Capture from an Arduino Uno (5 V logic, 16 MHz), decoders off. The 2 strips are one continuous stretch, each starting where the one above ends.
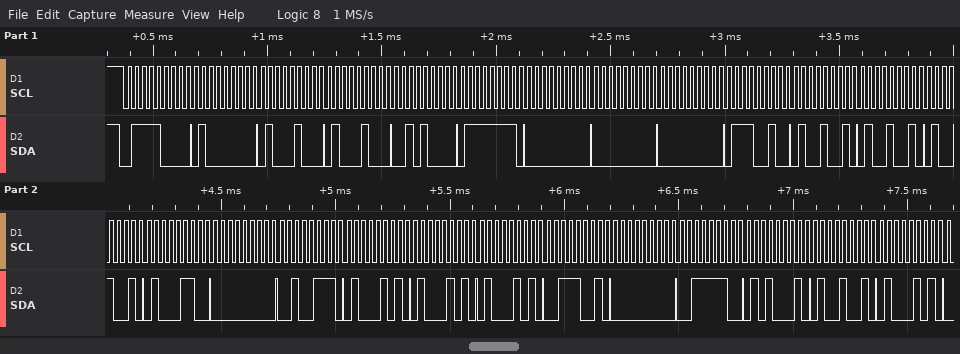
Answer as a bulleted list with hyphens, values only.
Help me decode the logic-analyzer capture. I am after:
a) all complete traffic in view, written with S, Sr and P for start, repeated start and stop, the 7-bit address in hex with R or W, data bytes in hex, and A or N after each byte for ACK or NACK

- S 3CW A 40 A 44 A 44 A 28 A 7F A 00 A 00 A 00 A 72 A 49 A 49 A 49 A 46 A 00 A 27 A 45 A 45 A 45 A 39 A 00 A 3E A 51 A 49 A 45 A
